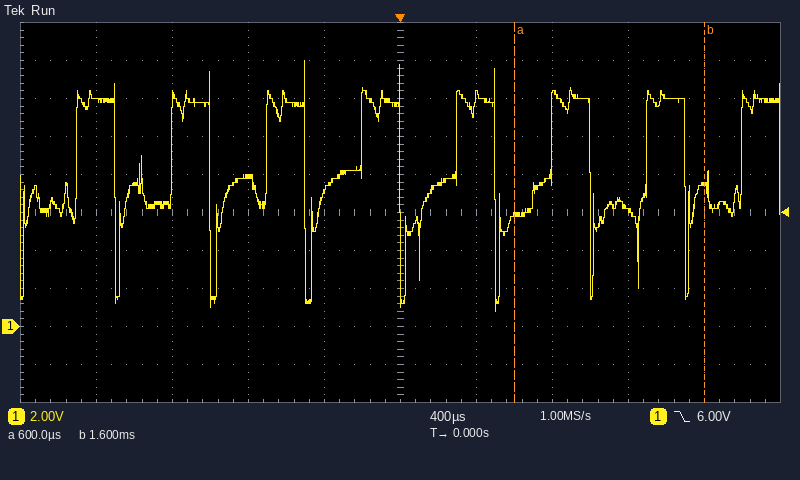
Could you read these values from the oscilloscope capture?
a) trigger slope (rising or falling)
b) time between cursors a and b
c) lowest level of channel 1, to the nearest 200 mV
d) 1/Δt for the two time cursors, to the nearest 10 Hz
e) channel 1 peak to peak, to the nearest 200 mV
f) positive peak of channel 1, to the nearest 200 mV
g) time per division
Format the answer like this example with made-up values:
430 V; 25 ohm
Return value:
falling; 1.00 ms; 800 mV; 1.00 kHz; 13.2 V; 14.0 V; 400 µs
